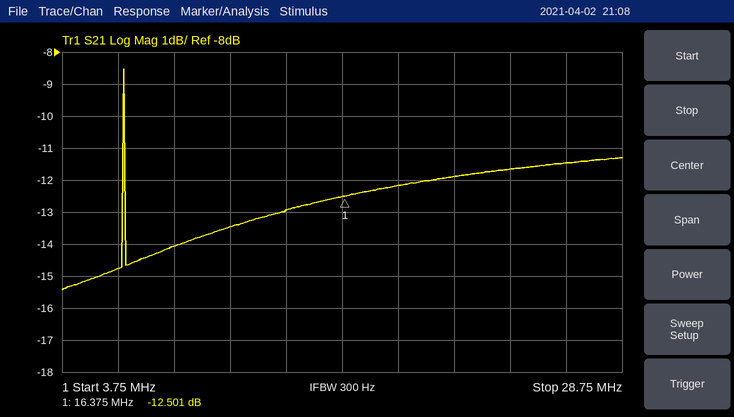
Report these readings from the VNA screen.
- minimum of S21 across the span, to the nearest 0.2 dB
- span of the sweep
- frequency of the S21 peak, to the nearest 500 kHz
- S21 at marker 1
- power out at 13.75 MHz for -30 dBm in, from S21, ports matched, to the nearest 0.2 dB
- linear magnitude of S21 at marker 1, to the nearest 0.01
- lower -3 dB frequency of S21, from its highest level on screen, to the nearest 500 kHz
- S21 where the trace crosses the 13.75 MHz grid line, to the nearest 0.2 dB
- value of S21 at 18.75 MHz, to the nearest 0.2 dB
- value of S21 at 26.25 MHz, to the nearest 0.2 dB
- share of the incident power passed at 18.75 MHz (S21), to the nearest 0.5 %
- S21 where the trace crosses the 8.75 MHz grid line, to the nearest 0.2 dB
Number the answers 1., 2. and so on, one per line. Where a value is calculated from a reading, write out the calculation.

1. -15.4 dB
2. 25 MHz
3. 6.5 MHz
4. -12.501 dB
5. -30 dBm + (-13.0 dB) = -43.0 dBm
6. 10^(-12.501/20) ≈ 0.24
7. 6.5 MHz
8. -13.0 dB
9. -12.2 dB
10. -11.4 dB
11. 10^(-12.2/10) ≈ 6.0 %
12. -14.0 dB
